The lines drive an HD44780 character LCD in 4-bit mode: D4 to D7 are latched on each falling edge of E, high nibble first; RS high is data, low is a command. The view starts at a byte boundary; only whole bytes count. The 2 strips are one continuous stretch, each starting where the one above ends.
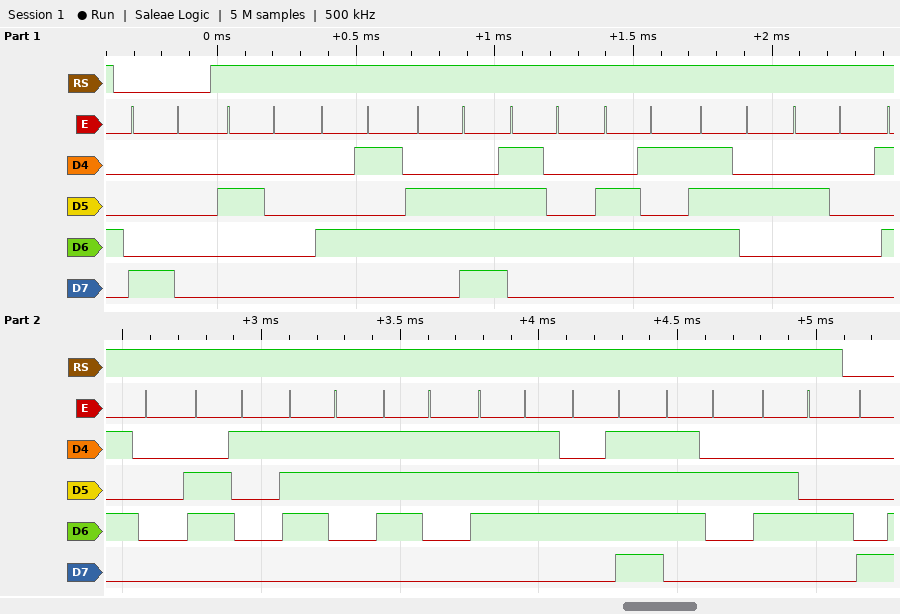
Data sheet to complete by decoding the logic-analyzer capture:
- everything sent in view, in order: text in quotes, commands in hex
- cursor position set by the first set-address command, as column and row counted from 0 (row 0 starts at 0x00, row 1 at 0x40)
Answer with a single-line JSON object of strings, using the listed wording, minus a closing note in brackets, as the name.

{"everything sent in view, in order: text in quotes, commands in hex": "0x80 \" Enter Password\"", "cursor position set by the first set-address command, as column and row counted from 0": "column 0, row 0"}
